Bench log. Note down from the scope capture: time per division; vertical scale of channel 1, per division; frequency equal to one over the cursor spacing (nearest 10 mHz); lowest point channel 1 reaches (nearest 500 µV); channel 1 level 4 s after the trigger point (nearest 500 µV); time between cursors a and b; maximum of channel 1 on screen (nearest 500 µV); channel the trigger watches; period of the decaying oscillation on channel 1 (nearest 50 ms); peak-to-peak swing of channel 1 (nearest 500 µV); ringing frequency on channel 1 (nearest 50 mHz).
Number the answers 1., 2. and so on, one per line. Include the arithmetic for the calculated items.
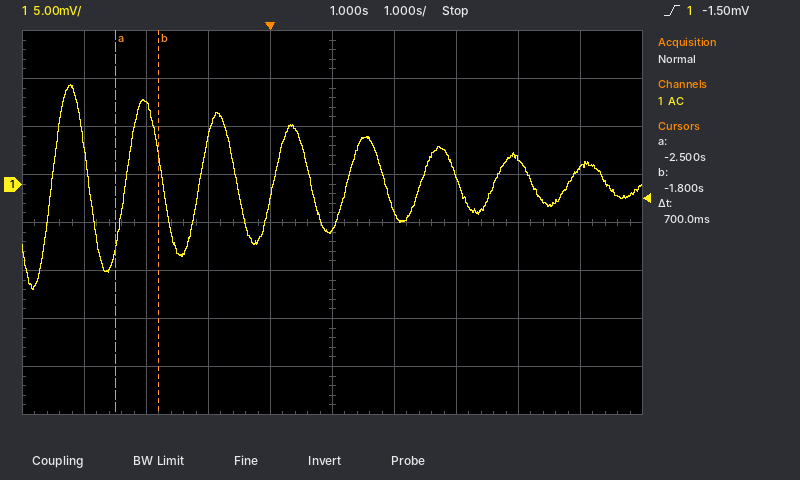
1. 1 s
2. 5 mV
3. 1 / 700 ms ≈ 1.43 Hz
4. -11.0 mV
5. 2.5 mV
6. 700 ms
7. 10.5 mV
8. channel 1
9. 1.20 s
10. 10.5 mV − (-11.0 mV) = 21.5 mV
11. 1 / 1.20 s ≈ 833 mHz, so 850 mHz to the nearest 50 mHz
